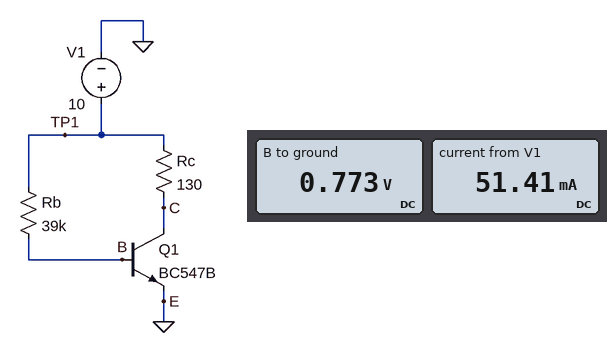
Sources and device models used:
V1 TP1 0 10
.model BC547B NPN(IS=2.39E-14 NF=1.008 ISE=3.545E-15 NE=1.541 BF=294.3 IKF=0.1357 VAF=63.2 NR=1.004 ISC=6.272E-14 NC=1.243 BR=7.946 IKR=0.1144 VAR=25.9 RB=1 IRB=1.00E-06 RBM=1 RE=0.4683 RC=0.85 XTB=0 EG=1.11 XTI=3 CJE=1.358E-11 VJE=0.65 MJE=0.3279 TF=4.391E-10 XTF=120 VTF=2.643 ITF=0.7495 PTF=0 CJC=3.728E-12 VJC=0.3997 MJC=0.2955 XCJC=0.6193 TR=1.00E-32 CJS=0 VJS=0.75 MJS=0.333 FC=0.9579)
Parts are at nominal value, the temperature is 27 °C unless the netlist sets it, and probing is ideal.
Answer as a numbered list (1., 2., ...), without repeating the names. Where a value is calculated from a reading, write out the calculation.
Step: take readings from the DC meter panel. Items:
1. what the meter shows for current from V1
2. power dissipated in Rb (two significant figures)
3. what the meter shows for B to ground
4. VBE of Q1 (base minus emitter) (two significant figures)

1. 51.41 mA
2. (10 V - 773 mV)^2 / 39 kΩ = 2.2 mW
3. 0.773 V
4. 773 mV = 770 mV
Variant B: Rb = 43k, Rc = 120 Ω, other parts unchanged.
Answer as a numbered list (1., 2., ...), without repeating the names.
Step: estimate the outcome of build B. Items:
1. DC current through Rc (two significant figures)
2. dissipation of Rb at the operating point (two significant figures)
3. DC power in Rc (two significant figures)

1. 48 mA
2. 2.0 mW
3. 280 mW
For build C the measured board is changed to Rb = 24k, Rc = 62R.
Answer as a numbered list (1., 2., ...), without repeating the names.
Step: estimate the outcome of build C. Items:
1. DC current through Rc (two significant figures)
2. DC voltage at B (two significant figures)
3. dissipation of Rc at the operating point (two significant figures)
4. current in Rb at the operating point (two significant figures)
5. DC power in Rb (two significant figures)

1. 76 mA
2. 800 mV
3. 360 mW
4. 380 µA
5. 3.5 mW
